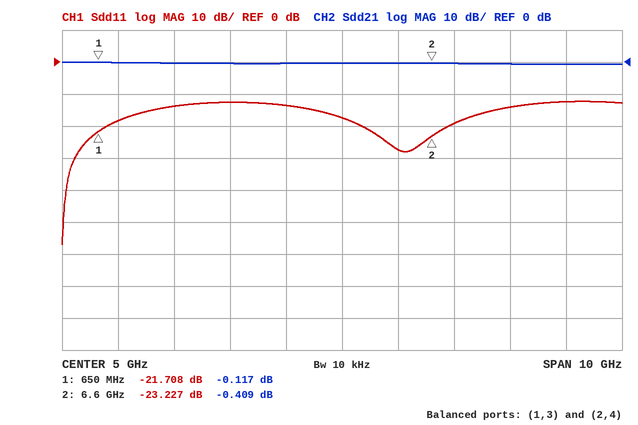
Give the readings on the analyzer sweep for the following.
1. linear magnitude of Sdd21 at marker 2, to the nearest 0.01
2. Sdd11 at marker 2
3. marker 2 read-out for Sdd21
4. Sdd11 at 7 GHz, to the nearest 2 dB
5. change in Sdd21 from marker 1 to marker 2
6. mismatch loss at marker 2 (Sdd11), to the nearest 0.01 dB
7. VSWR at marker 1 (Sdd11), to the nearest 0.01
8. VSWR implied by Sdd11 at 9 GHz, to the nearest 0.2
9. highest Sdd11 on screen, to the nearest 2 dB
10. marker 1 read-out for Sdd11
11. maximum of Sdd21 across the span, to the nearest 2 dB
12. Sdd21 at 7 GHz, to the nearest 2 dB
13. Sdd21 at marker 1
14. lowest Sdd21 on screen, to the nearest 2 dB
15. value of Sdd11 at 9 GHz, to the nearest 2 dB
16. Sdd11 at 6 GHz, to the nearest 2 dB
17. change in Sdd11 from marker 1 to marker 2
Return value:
0.95
-23.227 dB
-0.409 dB
-20 dB
-0.292 dB
0.02 dB
1.18
1.6
-12 dB
-21.708 dB
0 dB
0 dB
-0.117 dB
0 dB
-12 dB
-28 dB
-1.519 dB
